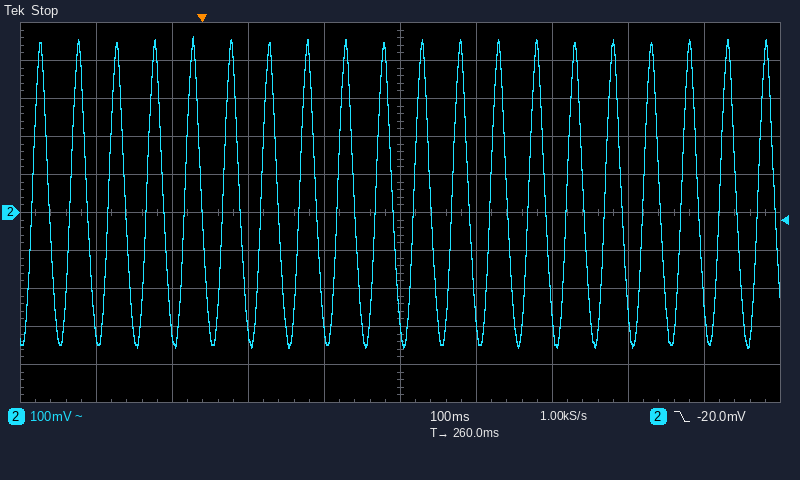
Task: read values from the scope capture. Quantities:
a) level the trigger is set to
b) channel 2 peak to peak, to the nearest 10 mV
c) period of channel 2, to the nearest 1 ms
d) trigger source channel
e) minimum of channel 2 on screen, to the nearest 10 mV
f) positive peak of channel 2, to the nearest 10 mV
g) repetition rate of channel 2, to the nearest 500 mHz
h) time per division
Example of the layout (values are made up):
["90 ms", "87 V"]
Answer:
["-20.0 mV", "820 mV", "50 ms", "channel 2", "-360 mV", "460 mV", "20.0 Hz", "100 ms"]
